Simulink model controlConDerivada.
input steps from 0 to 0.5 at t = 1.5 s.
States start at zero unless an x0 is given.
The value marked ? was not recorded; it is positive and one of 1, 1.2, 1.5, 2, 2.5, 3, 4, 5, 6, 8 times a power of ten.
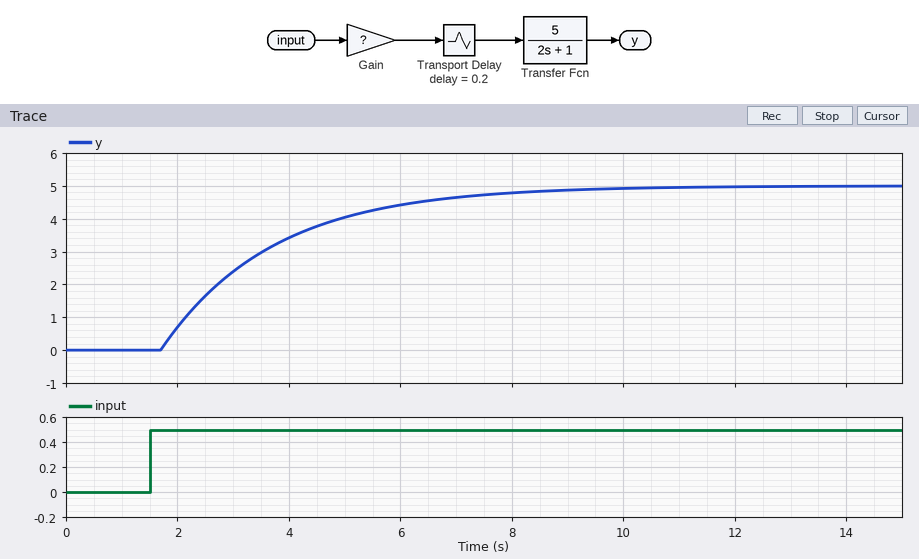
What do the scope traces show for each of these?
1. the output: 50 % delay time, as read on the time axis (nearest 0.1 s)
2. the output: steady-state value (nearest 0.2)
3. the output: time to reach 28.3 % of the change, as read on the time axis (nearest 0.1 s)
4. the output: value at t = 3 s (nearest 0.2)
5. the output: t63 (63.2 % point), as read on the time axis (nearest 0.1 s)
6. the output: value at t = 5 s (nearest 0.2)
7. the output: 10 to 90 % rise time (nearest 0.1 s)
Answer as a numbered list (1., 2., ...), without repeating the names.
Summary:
1. 3.1 s
2. 5.0
3. 2.4 s
4. 2.4
5. 3.7 s
6. 4.0
7. 4.4 s
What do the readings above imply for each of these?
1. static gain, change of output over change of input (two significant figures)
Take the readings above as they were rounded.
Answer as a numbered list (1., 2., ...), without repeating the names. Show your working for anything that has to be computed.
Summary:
1. (5 - 0) / (0.5 - 0) = 10
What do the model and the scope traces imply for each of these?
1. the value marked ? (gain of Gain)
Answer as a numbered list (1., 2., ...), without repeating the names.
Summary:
1. 2
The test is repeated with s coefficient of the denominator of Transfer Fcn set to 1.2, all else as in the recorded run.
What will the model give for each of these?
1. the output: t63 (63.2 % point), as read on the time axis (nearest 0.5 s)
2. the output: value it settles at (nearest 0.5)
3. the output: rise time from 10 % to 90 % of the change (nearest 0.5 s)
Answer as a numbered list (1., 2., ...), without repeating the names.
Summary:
1. 3.0 s
2. 5.0
3. 2.5 s
